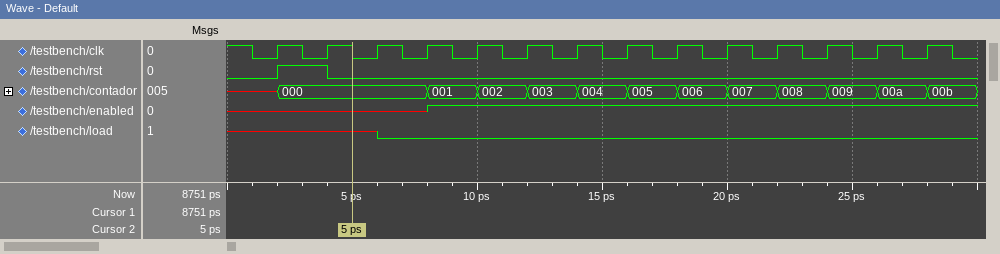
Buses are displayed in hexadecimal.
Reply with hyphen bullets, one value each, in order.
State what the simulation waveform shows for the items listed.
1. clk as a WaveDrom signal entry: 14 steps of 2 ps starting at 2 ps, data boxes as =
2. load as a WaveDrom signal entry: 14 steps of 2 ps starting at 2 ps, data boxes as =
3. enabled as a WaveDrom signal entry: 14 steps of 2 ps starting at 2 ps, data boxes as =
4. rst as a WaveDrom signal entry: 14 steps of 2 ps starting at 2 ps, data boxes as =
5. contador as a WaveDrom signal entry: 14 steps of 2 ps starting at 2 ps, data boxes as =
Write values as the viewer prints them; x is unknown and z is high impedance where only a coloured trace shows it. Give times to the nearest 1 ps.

- {name: 'clk', wave: 'p.............'}
- {name: 'load', wave: 'x.0...........'}
- {name: 'enabled', wave: 'x..1..........'}
- {name: 'rst', wave: '10............'}
- {name: 'contador', wave: '=..===========', data: '000 001 002 003 004 005 006 007 008 009 00a 00b'}
